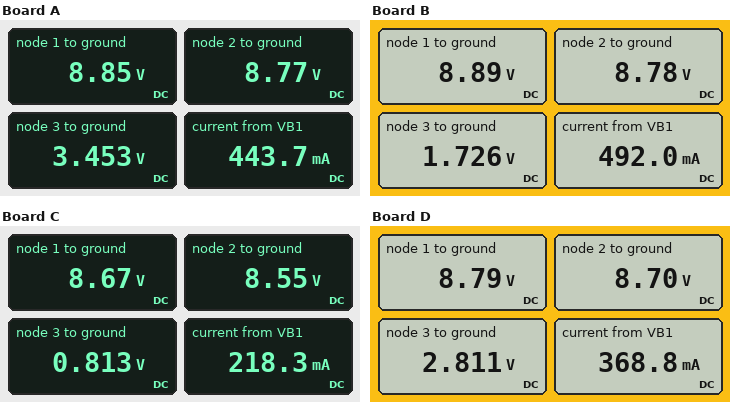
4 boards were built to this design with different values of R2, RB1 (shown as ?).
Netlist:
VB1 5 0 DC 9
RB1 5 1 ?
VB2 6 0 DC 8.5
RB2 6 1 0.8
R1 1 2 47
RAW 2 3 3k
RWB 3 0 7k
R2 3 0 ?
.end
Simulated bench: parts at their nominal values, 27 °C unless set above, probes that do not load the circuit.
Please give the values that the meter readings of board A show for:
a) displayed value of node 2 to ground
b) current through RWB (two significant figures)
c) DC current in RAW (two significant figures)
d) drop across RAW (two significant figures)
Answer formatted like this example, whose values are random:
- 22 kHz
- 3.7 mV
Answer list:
- 8.77 V
- 490 µA
- 1.8 mA
- 5.3 V
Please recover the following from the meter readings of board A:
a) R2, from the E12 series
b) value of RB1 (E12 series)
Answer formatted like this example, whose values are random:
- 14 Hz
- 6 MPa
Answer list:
- 2.7 kΩ
- 0.33 Ω
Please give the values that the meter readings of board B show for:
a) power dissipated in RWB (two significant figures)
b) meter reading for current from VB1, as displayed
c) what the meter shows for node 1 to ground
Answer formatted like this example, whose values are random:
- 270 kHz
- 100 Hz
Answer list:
- 430 µW
- 492.0 mA
- 8.89 V
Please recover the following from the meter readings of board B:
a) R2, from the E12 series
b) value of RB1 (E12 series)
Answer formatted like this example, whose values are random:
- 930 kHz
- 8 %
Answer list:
- 820 Ω
- 0.22 Ω
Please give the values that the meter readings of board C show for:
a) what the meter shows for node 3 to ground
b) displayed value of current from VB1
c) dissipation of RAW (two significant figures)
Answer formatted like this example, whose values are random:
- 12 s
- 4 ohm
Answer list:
- 0.813 V
- 218.3 mA
- 20 mW
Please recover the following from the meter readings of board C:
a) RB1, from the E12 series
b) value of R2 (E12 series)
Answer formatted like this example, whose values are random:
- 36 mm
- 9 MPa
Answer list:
- 1.5 Ω
- 330 Ω
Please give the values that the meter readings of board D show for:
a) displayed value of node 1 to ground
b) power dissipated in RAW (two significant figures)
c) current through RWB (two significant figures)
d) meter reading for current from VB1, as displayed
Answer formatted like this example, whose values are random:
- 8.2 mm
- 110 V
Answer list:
- 8.79 V
- 12 mW
- 400 µA
- 368.8 mA
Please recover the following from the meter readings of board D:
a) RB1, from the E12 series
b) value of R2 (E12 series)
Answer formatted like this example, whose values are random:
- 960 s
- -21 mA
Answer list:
- 0.56 Ω
- 1.8 kΩ
